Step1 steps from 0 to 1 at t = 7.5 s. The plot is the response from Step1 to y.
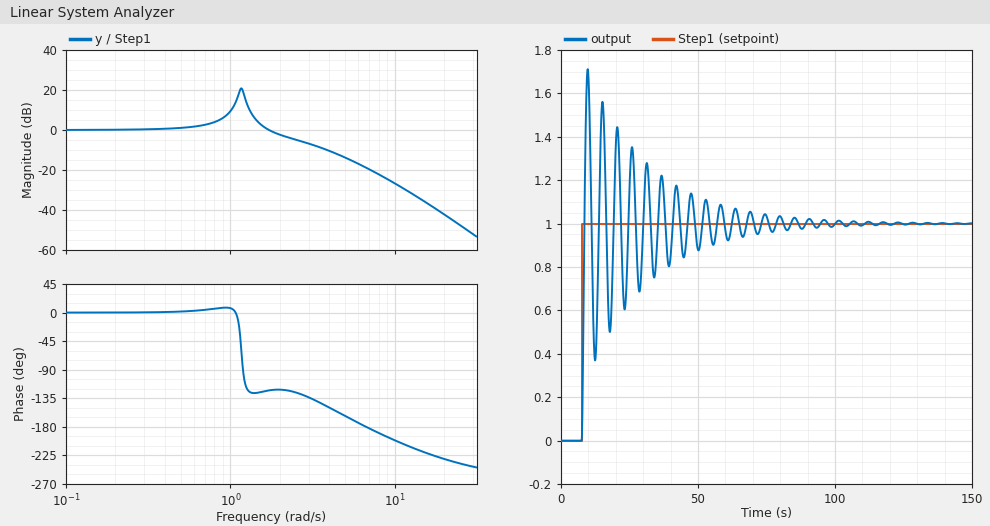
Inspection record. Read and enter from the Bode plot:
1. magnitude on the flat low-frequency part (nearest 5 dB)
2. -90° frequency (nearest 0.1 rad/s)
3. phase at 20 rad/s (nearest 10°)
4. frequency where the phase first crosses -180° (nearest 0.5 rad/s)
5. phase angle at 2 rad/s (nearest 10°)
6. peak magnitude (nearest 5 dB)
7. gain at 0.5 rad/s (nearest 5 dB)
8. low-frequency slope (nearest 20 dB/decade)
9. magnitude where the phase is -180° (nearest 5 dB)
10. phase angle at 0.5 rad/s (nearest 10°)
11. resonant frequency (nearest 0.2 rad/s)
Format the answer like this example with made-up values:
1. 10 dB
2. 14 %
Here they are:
1. 0 dB
2. 1.2 rad/s
3. -230°
4. 6.5 rad/s
5. -120°
6. 20 dB
7. 0 dB
8. 0 dB/decade
9. -20 dB
10. 0°
11. 1.2 rad/s
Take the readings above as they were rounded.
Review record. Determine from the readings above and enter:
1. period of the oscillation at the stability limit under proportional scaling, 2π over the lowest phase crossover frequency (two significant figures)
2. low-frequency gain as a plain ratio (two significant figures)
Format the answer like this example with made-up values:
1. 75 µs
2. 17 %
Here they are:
1. 0.97 s
2. 1.0
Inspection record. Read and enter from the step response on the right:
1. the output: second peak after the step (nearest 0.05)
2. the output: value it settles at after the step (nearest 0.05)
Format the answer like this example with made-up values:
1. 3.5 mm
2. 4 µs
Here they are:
1. 1.55
2. 1.00
